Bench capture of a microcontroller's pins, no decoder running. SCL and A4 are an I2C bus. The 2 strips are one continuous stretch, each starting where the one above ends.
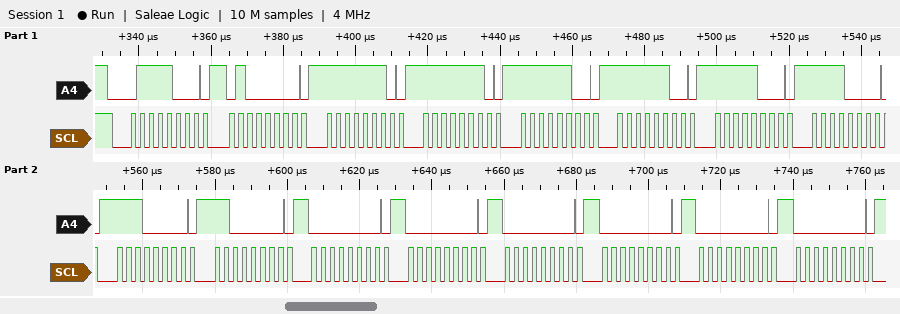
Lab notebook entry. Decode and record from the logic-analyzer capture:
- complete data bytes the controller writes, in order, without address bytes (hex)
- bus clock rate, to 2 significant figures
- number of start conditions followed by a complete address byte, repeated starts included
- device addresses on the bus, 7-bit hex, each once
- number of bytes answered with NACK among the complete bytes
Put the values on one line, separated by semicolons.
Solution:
40 FE FE FC FC F8 F0 E0 C0 00 00 00 00 00 00; 400 kHz; 1; 0x3C; 0
